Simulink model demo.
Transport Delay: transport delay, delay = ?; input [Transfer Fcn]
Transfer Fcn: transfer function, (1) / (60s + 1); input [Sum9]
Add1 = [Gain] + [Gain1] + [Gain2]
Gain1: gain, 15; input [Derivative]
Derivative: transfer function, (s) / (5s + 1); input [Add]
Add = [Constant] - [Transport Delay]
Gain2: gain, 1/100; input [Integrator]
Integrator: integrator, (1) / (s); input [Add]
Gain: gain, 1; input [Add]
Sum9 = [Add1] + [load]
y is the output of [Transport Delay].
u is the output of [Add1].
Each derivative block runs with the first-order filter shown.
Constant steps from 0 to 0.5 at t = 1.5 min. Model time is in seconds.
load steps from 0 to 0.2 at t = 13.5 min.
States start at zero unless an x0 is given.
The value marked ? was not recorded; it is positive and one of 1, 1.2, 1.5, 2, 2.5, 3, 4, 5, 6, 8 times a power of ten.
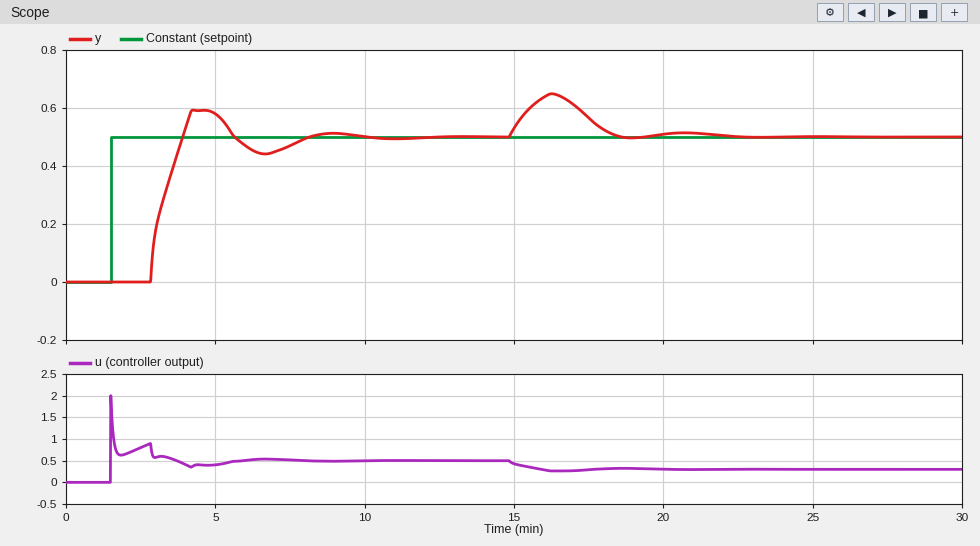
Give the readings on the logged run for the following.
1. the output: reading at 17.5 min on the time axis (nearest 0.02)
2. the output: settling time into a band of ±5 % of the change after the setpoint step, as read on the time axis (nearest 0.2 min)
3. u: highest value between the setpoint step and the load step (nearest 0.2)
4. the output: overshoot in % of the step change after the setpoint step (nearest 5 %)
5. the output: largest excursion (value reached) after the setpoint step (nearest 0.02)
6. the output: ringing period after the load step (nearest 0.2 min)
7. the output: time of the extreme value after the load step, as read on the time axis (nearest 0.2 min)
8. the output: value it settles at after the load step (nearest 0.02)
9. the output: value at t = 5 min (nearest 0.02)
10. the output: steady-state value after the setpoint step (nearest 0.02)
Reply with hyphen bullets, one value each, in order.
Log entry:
- 0.56
- 7.6 min
- 2.0
- 20 %
- 0.60
- 4.4 min
- 16.2 min
- 0.50
- 0.58
- 0.50
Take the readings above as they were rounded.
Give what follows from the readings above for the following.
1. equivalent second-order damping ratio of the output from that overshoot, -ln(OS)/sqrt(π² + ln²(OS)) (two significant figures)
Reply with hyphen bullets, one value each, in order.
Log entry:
- 0.46
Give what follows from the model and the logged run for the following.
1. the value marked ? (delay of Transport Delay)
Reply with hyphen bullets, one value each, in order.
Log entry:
- 80
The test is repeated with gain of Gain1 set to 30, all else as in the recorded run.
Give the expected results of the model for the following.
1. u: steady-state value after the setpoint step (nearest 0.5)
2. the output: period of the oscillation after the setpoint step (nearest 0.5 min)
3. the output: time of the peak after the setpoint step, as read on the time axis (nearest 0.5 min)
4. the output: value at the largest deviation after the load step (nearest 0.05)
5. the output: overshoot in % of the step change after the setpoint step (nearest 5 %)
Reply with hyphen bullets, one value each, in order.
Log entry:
- 0.5
- 3.0 min
- 4.0 min
- 0.65
- 25 %
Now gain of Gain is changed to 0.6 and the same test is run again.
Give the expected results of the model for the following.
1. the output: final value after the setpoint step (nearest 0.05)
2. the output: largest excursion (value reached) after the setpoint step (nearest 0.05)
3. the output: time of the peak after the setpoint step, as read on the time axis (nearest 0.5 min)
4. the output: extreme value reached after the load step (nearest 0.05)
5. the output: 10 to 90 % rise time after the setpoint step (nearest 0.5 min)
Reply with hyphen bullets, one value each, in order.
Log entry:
- 0.50
- 0.55
- 6.5 min
- 0.65
- 1.5 min
